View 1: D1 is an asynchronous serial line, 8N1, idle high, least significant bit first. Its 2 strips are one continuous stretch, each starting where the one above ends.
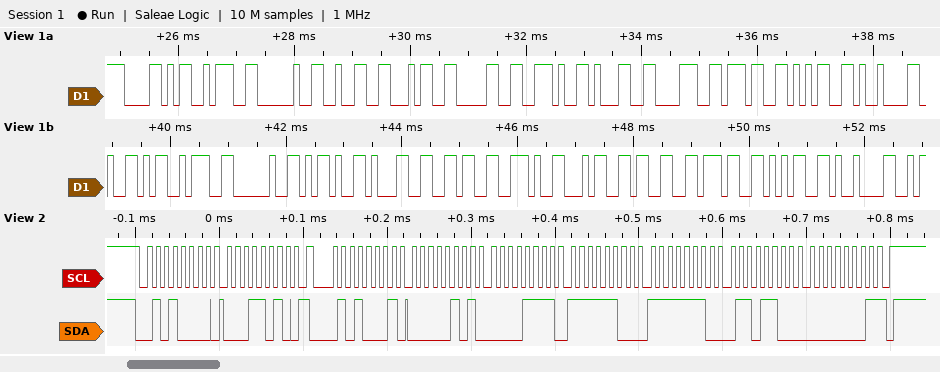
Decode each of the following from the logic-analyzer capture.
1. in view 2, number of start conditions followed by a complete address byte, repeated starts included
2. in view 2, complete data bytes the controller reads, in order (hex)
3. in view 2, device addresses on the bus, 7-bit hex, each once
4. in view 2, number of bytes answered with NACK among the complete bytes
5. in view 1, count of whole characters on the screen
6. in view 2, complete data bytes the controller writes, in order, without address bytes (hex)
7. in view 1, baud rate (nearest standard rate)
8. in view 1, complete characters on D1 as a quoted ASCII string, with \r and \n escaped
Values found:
2
05 0F FC FE 6C 01
0x28
1
24
1A
9600 baud
"X: 240.1875\tY: -16.4375\t"
